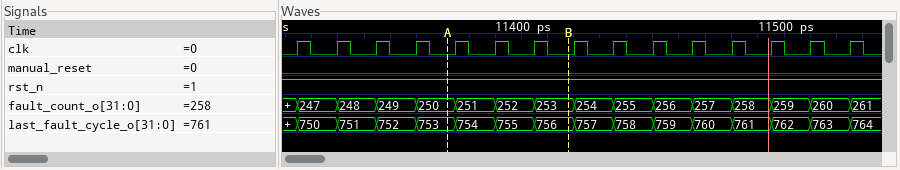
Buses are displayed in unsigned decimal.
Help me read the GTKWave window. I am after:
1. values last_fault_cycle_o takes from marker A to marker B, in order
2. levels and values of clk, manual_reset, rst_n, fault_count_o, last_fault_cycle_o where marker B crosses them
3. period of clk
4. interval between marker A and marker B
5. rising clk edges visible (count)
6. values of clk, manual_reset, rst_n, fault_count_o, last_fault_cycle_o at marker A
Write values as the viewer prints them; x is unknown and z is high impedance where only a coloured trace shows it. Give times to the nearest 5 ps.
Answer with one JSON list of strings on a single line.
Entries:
["753, 754, 755, 756", "clk=0, manual_reset=0, rst_n=1, fault_count_o=253, last_fault_cycle_o=756", "15 ps", "45 ps", "15", "clk=0, manual_reset=0, rst_n=1, fault_count_o=250, last_fault_cycle_o=753"]
